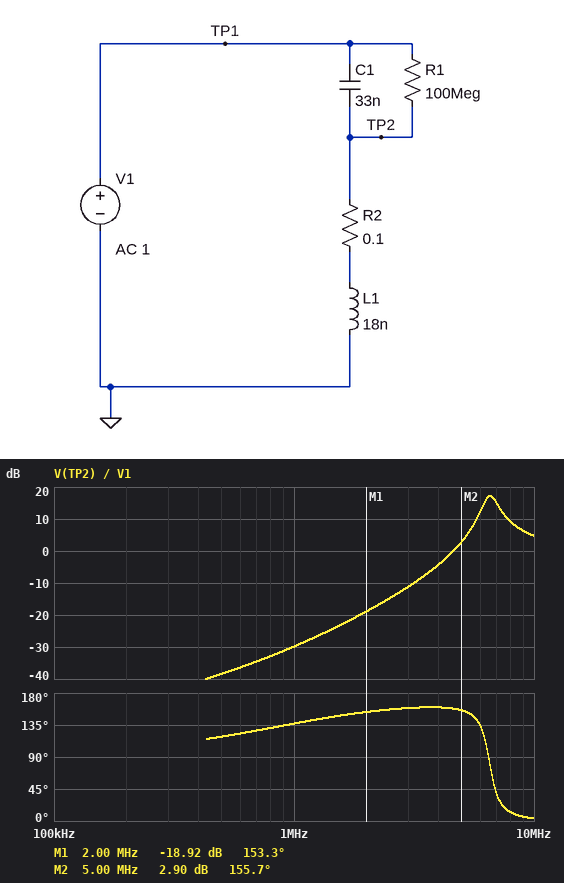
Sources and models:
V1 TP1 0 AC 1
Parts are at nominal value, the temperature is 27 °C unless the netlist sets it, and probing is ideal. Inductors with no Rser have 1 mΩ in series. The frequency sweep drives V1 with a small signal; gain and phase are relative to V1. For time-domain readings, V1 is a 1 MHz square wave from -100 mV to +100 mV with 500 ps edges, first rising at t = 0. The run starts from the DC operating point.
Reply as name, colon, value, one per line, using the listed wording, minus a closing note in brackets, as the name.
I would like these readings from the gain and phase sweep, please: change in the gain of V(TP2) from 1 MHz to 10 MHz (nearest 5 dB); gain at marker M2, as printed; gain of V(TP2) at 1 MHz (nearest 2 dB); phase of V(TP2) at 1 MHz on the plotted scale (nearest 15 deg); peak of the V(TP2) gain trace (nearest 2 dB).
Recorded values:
change in the gain of V(TP2) from 1 MHz to 10 MHz: 35 dB
gain at marker M2, as printed: 2.90 dB
gain of V(TP2) at 1 MHz: -30 dB
phase of V(TP2) at 1 MHz on the plotted scale: 135 deg
peak of the V(TP2) gain trace: 18 dB
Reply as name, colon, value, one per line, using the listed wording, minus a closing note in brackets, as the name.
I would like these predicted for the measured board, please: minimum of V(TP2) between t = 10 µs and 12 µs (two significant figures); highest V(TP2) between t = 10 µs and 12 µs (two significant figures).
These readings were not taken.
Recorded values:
minimum of V(TP2) between t = 10 µs and 12 µs: -190 mV
highest V(TP2) between t = 10 µs and 12 µs: 190 mV
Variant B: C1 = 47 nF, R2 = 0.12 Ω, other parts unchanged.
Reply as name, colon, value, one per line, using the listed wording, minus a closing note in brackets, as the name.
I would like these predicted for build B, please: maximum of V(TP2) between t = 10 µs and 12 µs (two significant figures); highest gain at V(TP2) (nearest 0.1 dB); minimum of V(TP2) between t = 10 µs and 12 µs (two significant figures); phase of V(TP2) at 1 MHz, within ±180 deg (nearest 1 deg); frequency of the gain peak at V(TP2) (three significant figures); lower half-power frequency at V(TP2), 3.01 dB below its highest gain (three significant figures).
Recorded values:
maximum of V(TP2) between t = 10 µs and 12 µs: 200 mV
highest gain at V(TP2): 14.4 dB
minimum of V(TP2) between t = 10 µs and 12 µs: -200 mV
phase of V(TP2) at 1 MHz, within ±180 deg: 131 deg
frequency of the gain peak at V(TP2): 5.52 MHz
lower half-power frequency at V(TP2), 3.01 dB below its highest gain: 5.04 MHz
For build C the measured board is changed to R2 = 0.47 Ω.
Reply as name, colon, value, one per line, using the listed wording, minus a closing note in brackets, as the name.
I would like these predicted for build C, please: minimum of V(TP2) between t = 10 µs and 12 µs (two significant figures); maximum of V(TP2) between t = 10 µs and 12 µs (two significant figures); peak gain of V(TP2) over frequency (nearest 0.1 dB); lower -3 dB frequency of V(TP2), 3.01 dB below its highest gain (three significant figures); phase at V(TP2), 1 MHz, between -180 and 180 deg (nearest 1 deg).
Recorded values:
minimum of V(TP2) between t = 10 µs and 12 µs: -200 mV
maximum of V(TP2) between t = 10 µs and 12 µs: 200 mV
peak gain of V(TP2) over frequency: 5.6 dB
lower -3 dB frequency of V(TP2), 3.01 dB below its highest gain: 5.30 MHz
phase at V(TP2), 1 MHz, between -180 and 180 deg: 98 deg
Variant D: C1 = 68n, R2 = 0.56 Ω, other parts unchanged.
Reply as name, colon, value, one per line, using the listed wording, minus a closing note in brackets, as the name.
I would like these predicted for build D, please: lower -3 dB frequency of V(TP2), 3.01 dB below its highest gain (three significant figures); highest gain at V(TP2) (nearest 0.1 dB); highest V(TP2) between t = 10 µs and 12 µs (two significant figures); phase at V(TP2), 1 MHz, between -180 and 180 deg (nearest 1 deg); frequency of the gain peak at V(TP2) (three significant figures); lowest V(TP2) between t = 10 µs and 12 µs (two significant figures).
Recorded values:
lower -3 dB frequency of V(TP2), 3.01 dB below its highest gain: 3.21 MHz
highest gain at V(TP2): 3.0 dB
highest V(TP2) between t = 10 µs and 12 µs: 200 mV
phase at V(TP2), 1 MHz, between -180 and 180 deg: 87 deg
frequency of the gain peak at V(TP2): 5.42 MHz
lowest V(TP2) between t = 10 µs and 12 µs: -200 mV
